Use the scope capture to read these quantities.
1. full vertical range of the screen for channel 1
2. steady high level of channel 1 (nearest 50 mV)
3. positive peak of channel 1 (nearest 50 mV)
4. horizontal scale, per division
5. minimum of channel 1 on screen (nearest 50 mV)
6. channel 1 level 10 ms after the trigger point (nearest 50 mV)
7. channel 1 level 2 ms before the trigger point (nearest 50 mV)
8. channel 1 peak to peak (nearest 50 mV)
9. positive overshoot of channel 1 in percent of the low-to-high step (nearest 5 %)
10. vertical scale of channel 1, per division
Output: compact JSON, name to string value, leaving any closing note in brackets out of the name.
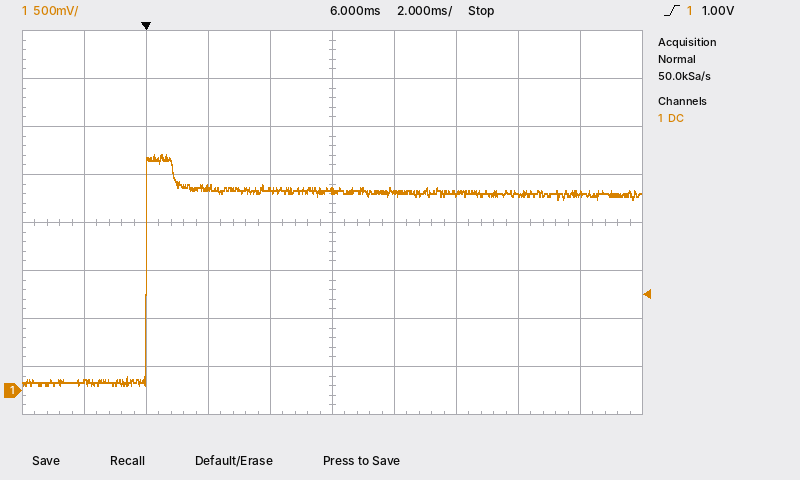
{"full vertical range of the screen for channel 1": "4 V", "steady high level of channel 1": "2.05 V", "positive peak of channel 1": "2.45 V", "horizontal scale, per division": "2 ms", "minimum of channel 1 on screen": "50 mV", "channel 1 level 10 ms after the trigger point": "2.05 V", "channel 1 level 2 ms before the trigger point": "100 mV", "channel 1 peak to peak": "2.40 V", "positive overshoot of channel 1 in percent of the low-to-high step": "20 %", "vertical scale of channel 1, per division": "500 mV"}
